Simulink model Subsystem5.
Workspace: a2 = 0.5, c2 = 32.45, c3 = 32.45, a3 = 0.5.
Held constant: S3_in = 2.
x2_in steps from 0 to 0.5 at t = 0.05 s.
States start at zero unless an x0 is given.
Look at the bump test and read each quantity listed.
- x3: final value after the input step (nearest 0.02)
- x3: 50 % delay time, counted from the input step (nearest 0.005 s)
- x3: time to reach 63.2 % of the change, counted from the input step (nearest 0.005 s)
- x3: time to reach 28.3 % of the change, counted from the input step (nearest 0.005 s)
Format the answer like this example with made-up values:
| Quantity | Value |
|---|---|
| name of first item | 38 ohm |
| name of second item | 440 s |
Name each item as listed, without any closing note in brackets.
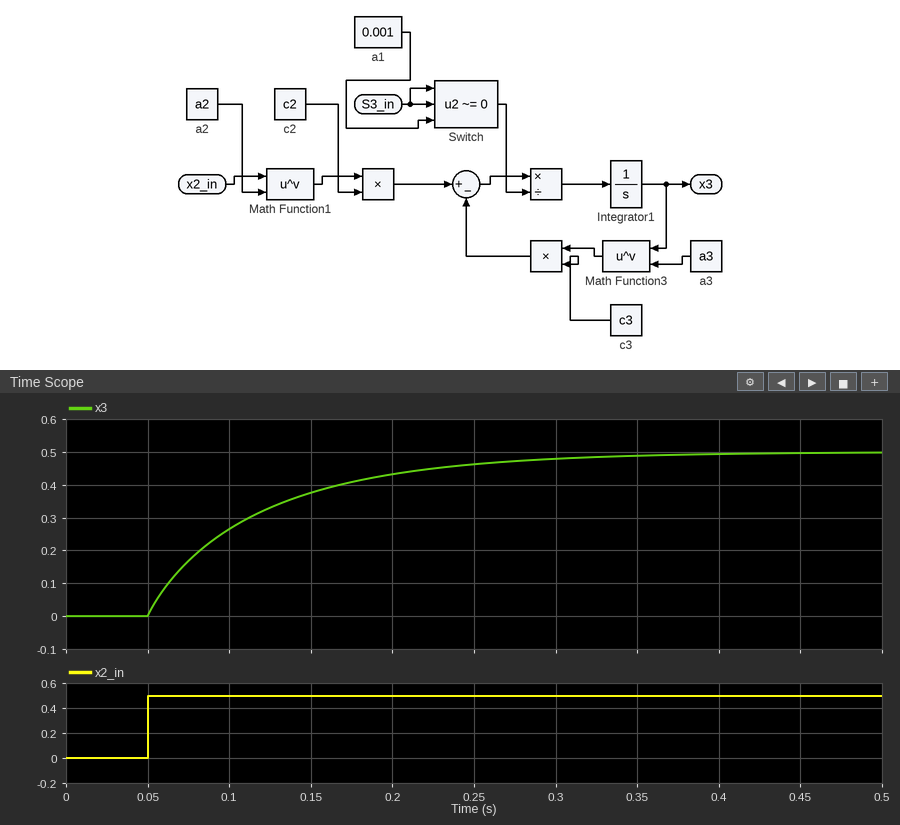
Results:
| Quantity | Value |
|---|---|
| x3: final value after the input step | 0.50 |
| x3: 50 % delay time, counted from the input step | 0.045 s |
| x3: time to reach 63.2 % of the change, counted from the input step | 0.070 s |
| x3: time to reach 28.3 % of the change, counted from the input step | 0.020 s |
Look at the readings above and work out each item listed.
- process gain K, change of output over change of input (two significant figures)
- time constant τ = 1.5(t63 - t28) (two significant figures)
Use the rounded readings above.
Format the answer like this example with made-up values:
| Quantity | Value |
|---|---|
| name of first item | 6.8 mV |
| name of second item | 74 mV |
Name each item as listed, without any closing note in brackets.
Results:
| Quantity | Value |
|---|---|
| process gain K, change of output over change of input | 1.0 |
| time constant τ = 1.5(t63 - t28) | 0.075 s |
